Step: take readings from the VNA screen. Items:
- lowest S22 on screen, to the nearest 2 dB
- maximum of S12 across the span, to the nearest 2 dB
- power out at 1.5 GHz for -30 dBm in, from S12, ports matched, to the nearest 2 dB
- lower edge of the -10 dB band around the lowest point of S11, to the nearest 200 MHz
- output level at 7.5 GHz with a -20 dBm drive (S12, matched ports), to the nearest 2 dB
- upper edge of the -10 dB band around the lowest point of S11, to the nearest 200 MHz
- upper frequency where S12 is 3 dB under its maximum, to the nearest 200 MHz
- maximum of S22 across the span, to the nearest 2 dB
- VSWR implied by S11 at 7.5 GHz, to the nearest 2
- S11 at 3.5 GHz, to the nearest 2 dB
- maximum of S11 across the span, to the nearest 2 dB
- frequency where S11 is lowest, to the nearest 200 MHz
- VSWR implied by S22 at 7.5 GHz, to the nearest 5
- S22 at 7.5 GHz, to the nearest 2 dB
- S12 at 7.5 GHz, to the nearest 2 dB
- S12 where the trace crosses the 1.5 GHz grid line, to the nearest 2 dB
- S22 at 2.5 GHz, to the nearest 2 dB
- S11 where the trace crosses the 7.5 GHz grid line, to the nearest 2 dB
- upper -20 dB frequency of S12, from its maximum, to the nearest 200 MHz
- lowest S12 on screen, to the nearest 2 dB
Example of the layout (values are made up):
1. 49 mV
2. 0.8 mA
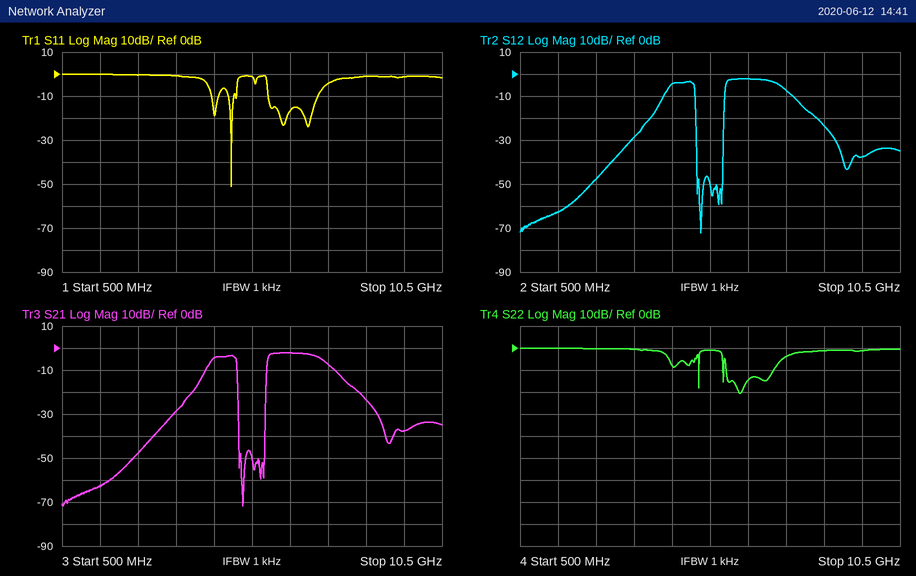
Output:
1. -20 dB
2. -2 dB
3. -92 dBm
4. 4.8 GHz
5. -28 dBm
6. 5.0 GHz
7. 7.4 GHz
8. 0 dB
9. 4
10. 0 dB
11. 0 dB
12. 5.0 GHz
13. 5
14. -4 dB
15. -8 dB
16. -62 dB
17. 0 dB
18. -4 dB
19. 8.4 GHz
20. -72 dB
